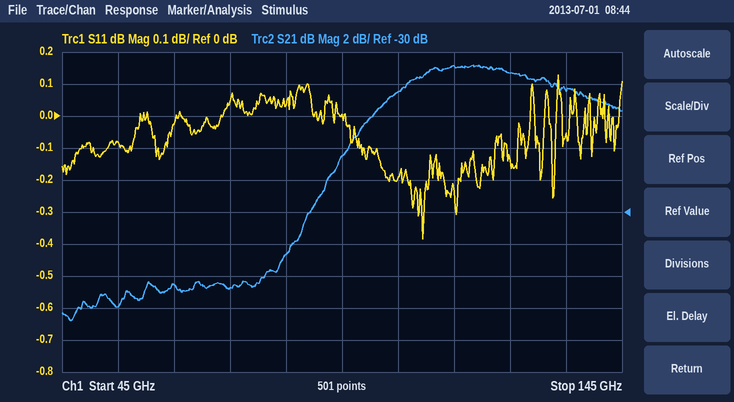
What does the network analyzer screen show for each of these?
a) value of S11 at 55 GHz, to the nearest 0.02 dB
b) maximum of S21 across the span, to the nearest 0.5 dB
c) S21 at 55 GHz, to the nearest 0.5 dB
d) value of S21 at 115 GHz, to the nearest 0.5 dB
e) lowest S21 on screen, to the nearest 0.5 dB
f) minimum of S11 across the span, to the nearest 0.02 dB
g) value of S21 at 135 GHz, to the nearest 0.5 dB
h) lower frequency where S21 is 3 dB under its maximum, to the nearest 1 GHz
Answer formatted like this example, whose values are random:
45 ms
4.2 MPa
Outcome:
-0.08 dB
-21.0 dB
-36.0 dB
-21.0 dB
-37.0 dB
-0.38 dB
-22.5 dB
101 GHz
